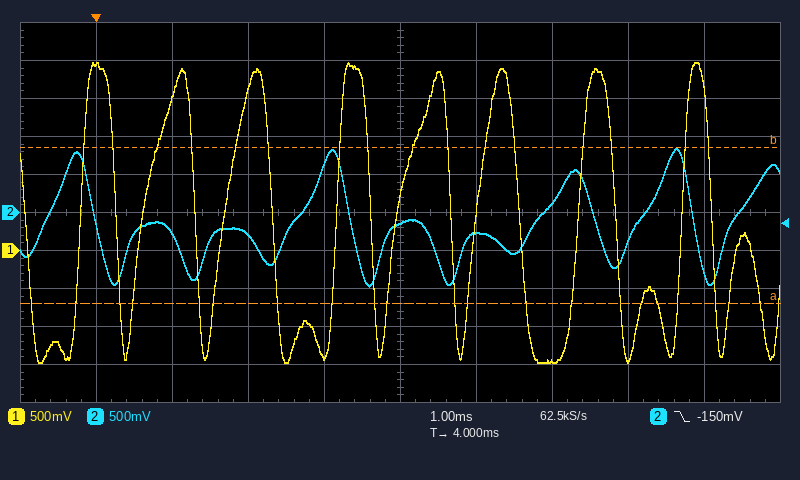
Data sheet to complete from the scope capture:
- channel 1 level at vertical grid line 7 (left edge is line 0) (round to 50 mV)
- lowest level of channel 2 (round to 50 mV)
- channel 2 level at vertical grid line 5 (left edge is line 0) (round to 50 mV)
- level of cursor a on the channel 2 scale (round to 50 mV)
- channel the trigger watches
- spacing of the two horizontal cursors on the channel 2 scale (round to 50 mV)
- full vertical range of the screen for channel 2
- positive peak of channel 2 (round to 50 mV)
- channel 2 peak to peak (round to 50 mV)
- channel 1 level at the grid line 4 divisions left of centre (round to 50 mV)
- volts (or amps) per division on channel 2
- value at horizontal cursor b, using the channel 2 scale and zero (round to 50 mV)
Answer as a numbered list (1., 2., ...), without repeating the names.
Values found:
1. -1.45 V
2. -950 mV
3. -150 mV
4. -1.20 V
5. channel 2
6. 2.05 V
7. 5 V
8. 850 mV
9. 1.80 V
10. 2.45 V
11. 500 mV
12. 850 mV
